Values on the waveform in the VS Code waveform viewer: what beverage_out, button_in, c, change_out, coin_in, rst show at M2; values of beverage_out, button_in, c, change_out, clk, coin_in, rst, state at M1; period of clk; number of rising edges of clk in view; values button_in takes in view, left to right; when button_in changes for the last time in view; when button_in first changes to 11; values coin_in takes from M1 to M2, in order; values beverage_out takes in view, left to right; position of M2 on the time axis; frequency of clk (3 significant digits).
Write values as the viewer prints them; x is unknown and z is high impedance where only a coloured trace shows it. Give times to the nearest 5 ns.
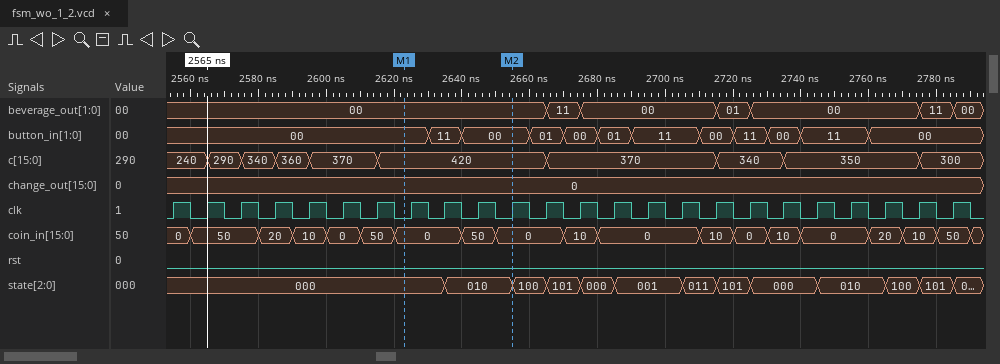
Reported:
beverage_out=00, button_in=00, c=420, change_out=0, coin_in=0, rst=0
beverage_out=00, button_in=00, c=420, change_out=0, clk=0, coin_in=0, rst=0, state=000
10 ns
24
00, 11, 00, 01, 00, 01, 11, 00, 11, 00, 11, 00
2760 ns
2630 ns
0, 50, 0
00, 11, 00, 01, 00, 11, 00
2655 ns
100 MHz
